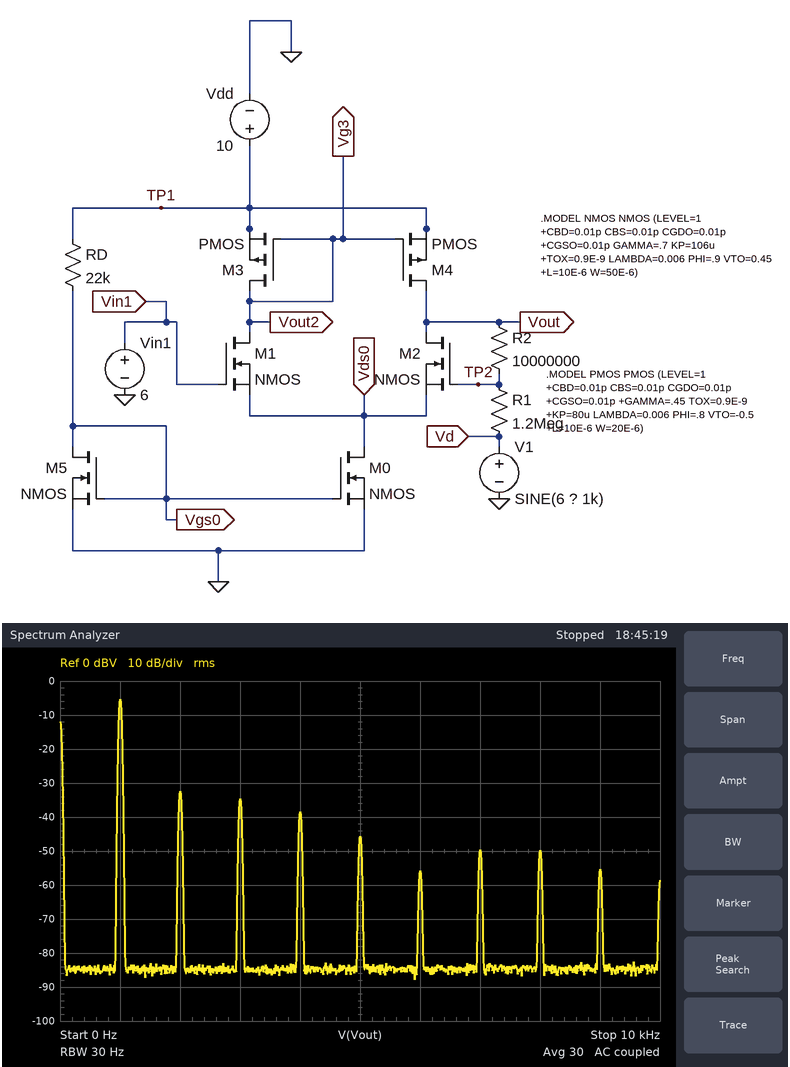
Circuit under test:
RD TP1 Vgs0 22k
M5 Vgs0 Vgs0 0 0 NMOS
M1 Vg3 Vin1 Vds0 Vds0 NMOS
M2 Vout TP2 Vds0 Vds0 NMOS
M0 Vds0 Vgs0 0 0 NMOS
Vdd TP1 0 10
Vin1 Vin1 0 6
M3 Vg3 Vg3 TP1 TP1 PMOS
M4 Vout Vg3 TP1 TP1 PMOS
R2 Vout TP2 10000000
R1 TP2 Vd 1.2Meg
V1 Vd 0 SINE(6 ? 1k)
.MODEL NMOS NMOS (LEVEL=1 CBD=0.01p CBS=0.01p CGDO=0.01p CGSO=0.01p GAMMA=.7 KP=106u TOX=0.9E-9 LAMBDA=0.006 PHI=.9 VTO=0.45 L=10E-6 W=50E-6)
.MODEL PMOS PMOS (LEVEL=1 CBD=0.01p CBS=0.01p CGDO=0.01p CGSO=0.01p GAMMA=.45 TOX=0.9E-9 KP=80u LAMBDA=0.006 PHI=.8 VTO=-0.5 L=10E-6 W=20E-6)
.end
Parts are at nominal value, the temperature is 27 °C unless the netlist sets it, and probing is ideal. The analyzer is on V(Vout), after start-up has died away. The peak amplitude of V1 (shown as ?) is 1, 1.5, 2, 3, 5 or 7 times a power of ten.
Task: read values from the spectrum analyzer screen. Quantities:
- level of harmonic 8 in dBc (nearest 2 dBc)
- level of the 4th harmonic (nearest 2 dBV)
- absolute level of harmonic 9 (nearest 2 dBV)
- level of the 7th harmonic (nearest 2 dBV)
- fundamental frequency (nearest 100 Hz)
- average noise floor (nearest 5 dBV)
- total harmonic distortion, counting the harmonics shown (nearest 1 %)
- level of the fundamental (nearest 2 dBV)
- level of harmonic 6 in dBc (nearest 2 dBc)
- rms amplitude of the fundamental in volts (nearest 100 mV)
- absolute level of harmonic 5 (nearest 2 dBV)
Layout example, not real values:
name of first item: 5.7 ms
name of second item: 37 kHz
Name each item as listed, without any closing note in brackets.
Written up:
level of harmonic 8 in dBc: -44 dBc
level of the 4th harmonic: -38 dBV
absolute level of harmonic 9: -56 dBV
level of the 7th harmonic: -50 dBV
fundamental frequency: 1.0 kHz
average noise floor: -85 dBV
total harmonic distortion, counting the harmonics shown: 6 %
level of the fundamental: -6 dBV
level of harmonic 6 in dBc: -50 dBc
rms amplitude of the fundamental in volts: 500 mV
absolute level of harmonic 5: -46 dBV
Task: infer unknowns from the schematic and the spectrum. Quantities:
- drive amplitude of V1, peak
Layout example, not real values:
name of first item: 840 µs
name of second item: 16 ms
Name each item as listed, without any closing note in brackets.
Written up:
drive amplitude of V1, peak: 100 mV
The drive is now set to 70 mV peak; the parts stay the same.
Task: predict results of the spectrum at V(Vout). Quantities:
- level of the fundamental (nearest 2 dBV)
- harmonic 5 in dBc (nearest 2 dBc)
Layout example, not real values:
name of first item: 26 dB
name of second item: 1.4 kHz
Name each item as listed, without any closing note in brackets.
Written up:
level of the fundamental: -8 dBV
harmonic 5 in dBc: -60 dBc
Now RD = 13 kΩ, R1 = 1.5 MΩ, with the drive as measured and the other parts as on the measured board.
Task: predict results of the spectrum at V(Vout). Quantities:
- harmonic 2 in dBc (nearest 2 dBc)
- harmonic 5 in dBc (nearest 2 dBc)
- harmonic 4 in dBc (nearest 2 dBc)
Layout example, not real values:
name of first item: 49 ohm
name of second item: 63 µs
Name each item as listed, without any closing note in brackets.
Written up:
harmonic 2 in dBc: -38 dBc
harmonic 5 in dBc: -42 dBc
harmonic 4 in dBc: -40 dBc
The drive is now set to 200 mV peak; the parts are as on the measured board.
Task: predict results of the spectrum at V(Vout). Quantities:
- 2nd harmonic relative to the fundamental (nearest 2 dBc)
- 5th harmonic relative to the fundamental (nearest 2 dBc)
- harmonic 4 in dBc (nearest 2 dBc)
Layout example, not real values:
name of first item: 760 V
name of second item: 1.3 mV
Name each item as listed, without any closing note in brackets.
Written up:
2nd harmonic relative to the fundamental: -16 dBc
5th harmonic relative to the fundamental: -32 dBc
harmonic 4 in dBc: -42 dBc
